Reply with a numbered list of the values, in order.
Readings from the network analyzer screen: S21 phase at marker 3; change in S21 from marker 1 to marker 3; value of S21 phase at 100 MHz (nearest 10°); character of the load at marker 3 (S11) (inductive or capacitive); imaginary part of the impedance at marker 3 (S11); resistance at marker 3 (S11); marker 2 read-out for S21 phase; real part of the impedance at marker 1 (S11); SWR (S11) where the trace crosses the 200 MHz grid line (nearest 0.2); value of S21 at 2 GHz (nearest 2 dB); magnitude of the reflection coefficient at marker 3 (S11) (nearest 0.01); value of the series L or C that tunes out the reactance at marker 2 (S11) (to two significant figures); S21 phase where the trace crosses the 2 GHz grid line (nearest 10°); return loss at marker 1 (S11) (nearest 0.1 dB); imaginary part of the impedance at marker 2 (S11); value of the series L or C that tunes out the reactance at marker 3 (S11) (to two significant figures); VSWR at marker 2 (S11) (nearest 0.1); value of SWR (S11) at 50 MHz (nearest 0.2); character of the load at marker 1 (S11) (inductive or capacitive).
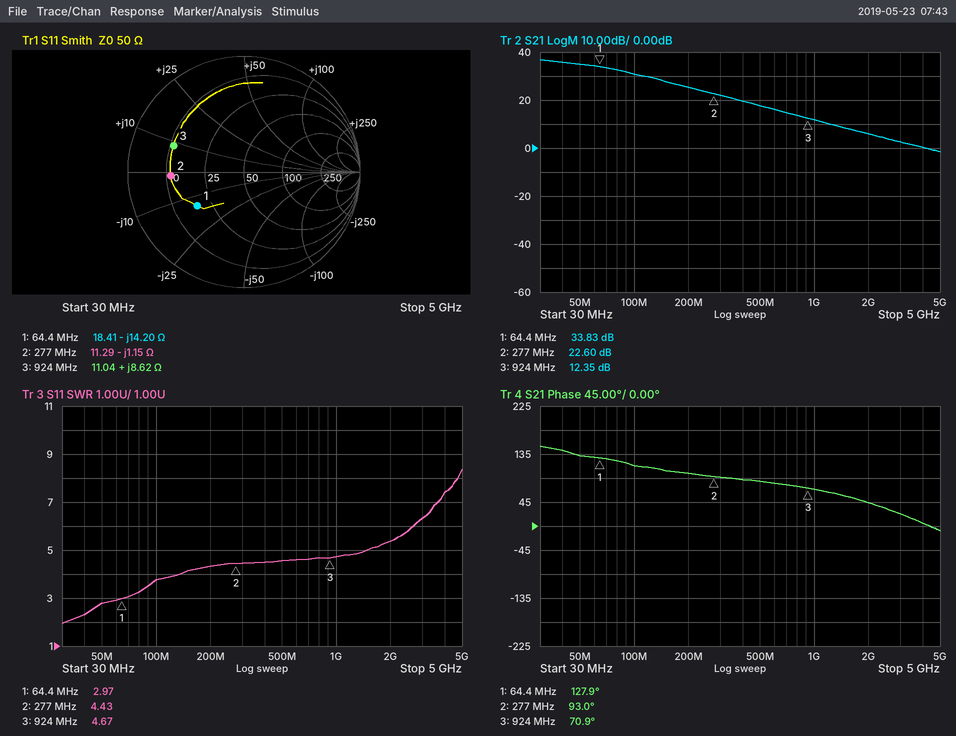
1. 70.9°
2. -21.48 dB
3. 110°
4. inductive
5. +8.62 Ω
6. 11.04 Ω
7. 93.0°
8. 18.41 Ω
9. 4.4
10. 6 dB
11. 0.65
12. 660 pH
13. 40°
14. 6.1 dB
15. -1.15 Ω
16. 20 pF
17. 4.4
18. 2.8
19. capacitive
